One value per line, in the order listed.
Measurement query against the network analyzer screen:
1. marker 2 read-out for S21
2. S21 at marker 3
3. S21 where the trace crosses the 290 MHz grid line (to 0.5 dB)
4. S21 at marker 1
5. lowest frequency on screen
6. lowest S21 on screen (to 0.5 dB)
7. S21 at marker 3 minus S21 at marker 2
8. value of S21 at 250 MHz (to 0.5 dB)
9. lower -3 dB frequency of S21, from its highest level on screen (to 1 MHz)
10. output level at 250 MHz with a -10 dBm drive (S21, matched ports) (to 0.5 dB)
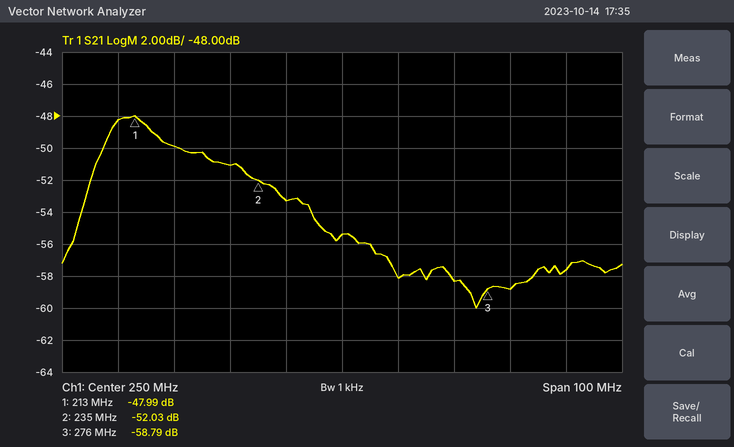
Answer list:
-52.03 dB
-58.79 dB
-57.5 dB
-47.99 dB
200 MHz
-60.0 dB
-6.76 dB
-55.5 dB
206 MHz
-65.5 dBm
